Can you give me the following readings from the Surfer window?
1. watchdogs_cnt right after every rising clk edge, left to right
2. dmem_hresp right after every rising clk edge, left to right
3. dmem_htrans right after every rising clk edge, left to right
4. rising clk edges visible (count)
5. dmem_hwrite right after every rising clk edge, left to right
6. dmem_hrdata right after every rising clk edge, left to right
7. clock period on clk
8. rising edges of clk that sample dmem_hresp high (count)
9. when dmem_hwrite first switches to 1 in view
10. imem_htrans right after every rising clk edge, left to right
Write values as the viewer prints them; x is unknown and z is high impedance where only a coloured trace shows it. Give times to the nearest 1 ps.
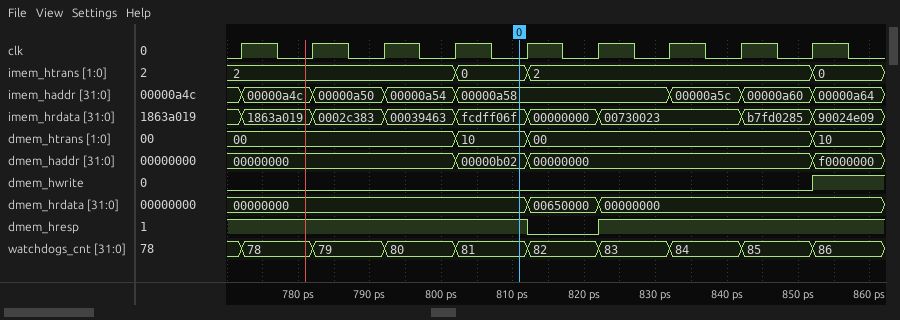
78, 79, 80, 81, 82, 83, 84, 85, 86
1 1 1 1 0 1 1 1 1
00, 00, 00, 10, 00, 00, 00, 00, 10
9
0 0 0 0 0 0 0 0 1
00000000, 00000000, 00000000, 00000000, 00650000, 00000000, 00000000, 00000000, 00000000
10 ps
8
852 ps
2, 2, 2, 0, 2, 2, 2, 2, 0
